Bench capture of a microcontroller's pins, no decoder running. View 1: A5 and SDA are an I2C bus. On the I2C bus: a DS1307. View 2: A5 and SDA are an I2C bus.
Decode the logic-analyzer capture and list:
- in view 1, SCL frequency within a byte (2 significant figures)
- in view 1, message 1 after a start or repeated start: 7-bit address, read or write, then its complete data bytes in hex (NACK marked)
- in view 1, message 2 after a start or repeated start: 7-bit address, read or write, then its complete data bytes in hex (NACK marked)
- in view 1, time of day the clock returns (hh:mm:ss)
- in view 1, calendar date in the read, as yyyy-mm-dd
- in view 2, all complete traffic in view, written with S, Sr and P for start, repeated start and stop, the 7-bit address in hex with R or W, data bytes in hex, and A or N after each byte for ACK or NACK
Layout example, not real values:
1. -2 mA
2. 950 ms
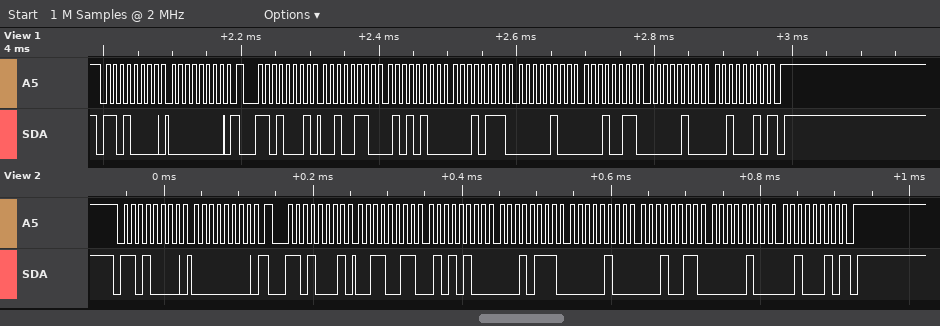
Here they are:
1. 100 kHz
2. 0x68 write: 00
3. 0x68 read: 26 54 17 04 13 04 22 NACK
4. 17:54:26
5. 2022-04-13
6. S 68W A 00 A Sr 68R A 33 A 54 A 17 A 04 A 13 A 04 A 22 N P
